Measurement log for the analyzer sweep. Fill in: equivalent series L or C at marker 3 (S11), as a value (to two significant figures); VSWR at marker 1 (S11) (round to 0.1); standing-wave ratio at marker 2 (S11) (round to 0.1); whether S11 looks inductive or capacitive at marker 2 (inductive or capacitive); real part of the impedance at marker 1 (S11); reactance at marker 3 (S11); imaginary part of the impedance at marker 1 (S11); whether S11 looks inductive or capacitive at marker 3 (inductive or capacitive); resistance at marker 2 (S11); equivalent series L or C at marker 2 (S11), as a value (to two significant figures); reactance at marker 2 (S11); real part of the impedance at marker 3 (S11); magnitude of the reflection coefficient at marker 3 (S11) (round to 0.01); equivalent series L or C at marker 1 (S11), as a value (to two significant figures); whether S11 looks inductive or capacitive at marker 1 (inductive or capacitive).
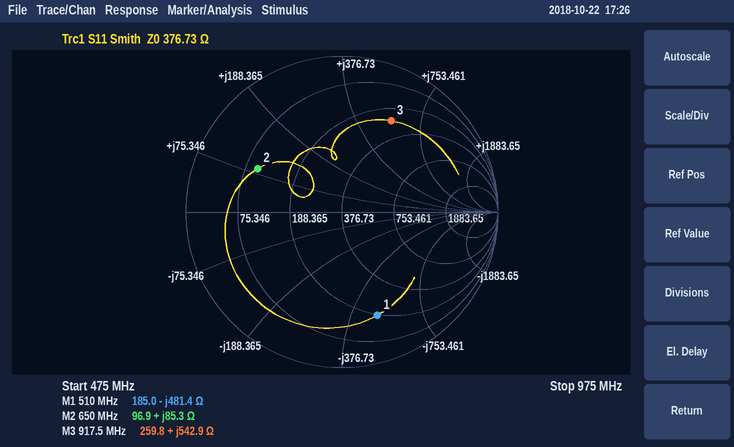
94 nH
5.7
4.1
inductive
185.0 Ω
+542.9 Ω
-481.4 Ω
inductive
96.9 Ω
21 nH
+85.3 Ω
259.8 Ω
0.66
650 fF
capacitive
